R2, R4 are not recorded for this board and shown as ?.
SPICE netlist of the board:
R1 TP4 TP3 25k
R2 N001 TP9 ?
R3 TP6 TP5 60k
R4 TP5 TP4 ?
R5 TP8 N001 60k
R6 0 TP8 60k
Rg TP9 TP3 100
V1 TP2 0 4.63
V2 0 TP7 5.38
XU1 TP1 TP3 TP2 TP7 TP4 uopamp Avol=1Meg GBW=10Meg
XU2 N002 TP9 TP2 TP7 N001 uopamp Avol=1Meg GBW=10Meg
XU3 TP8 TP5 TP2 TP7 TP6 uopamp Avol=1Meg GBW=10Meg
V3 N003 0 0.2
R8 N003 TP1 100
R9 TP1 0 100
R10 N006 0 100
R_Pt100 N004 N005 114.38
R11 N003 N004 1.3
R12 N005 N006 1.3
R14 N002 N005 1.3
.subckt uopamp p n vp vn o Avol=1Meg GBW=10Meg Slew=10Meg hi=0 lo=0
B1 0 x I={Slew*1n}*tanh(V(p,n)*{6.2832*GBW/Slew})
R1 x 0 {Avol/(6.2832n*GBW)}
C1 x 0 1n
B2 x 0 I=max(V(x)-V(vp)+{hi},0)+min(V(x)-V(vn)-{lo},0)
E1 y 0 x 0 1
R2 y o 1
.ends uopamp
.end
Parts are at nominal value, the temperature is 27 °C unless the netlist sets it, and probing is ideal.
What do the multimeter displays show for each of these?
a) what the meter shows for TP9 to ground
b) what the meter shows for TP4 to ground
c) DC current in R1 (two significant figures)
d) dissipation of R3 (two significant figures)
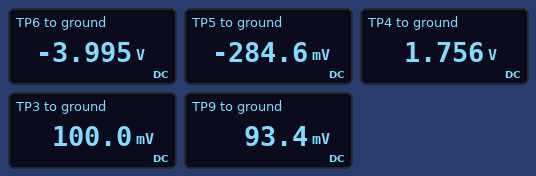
93.4 mV
1.756 V
66 µA
230 µW
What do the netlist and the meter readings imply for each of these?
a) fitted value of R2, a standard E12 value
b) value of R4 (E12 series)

10 kΩ
33 kΩ
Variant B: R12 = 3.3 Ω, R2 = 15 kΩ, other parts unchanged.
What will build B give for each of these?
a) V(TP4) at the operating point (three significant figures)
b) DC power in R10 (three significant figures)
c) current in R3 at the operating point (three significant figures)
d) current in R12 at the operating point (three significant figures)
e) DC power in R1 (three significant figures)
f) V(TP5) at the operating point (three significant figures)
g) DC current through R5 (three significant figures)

1.51 V
83.4 µW
57.3 µA
913 µA
79.8 µW
-377 mV
6.28 µA
